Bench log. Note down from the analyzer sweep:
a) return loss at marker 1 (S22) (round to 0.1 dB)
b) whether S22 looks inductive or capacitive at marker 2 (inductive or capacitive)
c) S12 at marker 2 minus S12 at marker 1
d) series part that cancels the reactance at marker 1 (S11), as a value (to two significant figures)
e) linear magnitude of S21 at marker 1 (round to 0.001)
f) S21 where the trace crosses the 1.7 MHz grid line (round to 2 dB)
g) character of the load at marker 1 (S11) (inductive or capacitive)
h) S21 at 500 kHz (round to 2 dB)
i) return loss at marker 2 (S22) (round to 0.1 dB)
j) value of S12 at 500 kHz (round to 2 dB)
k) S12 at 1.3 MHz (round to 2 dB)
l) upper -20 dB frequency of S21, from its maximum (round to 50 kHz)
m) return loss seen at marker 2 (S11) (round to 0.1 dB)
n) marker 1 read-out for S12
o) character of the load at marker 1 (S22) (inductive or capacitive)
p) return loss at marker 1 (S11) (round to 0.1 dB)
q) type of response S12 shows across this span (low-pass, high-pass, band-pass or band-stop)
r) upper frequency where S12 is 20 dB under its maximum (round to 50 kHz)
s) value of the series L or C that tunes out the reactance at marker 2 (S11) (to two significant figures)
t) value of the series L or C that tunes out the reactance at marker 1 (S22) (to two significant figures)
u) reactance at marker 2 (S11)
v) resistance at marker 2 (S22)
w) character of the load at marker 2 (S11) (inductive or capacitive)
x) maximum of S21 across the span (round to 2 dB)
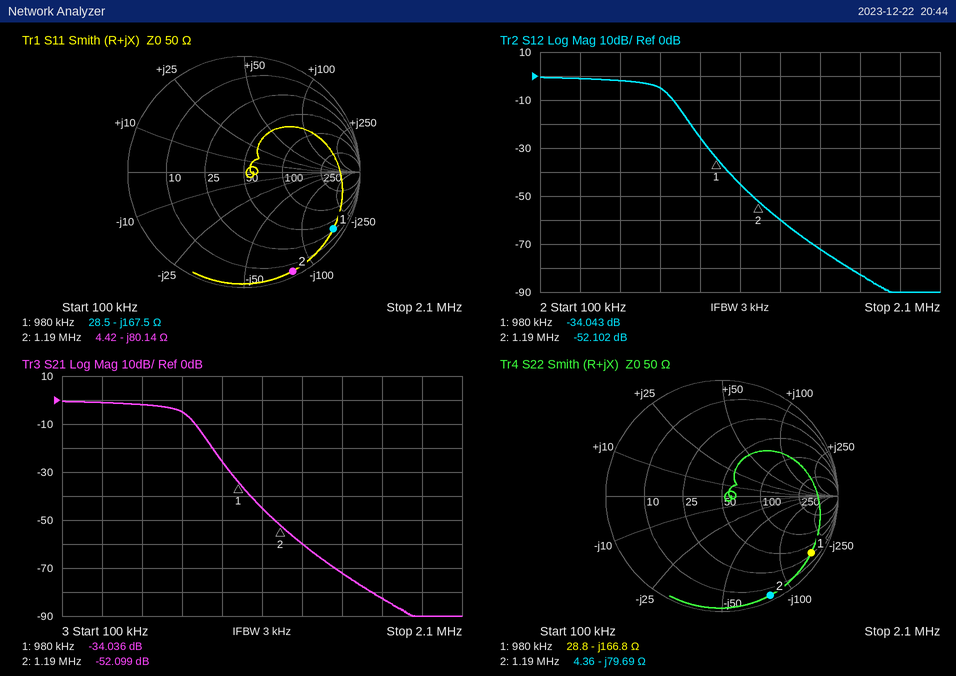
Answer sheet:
0.8 dB
capacitive
-18.059 dB
27 µH
0.020
-82 dB
capacitive
-2 dB
0.4 dB
-2 dB
-60 dB
850 kHz
0.4 dB
-34.043 dB
capacitive
0.8 dB
low-pass
850 kHz
11 µH
27 µH
-80.14 Ω
4.36 Ω
capacitive
0 dB
